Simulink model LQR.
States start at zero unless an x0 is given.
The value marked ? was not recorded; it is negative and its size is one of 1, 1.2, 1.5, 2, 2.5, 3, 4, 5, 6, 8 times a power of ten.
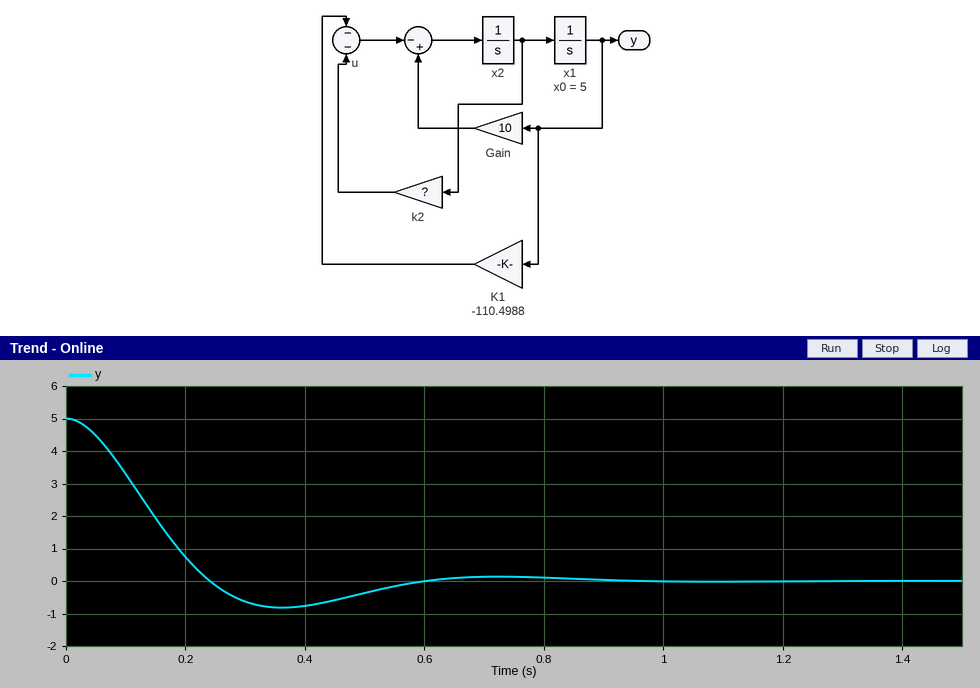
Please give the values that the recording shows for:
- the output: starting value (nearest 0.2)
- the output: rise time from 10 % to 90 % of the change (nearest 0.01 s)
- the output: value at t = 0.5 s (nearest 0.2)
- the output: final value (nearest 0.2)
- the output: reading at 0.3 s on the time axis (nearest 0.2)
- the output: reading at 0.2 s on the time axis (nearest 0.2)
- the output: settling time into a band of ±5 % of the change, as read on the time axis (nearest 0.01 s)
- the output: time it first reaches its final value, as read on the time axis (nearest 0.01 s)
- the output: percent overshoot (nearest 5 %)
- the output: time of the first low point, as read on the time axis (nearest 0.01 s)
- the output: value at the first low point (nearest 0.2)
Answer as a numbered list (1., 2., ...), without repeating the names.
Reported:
1. 5.0
2. 0.16 s
3. -0.4
4. 0.0
5. -0.6
6. 0.8
7. 0.53 s
8. 0.24 s
9. 15 %
10. 0.36 s
11. -0.8
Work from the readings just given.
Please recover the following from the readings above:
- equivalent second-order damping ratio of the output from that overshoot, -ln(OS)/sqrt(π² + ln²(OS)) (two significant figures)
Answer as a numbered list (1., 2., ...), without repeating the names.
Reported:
1. 0.52
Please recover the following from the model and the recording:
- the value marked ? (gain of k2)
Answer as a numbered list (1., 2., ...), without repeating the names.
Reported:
1. -10
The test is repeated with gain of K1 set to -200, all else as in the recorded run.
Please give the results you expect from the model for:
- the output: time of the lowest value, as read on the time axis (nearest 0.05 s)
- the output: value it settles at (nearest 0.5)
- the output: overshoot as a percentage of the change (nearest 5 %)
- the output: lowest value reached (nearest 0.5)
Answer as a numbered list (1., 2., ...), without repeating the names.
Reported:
1. 0.25 s
2. 0.0
3. 30 %
4. -1.5
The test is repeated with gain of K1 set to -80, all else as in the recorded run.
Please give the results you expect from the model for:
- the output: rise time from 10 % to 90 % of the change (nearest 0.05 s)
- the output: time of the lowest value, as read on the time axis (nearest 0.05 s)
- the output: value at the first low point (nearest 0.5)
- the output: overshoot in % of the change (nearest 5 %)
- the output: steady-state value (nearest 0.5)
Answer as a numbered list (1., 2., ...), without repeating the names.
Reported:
1. 0.20 s
2. 0.45 s
3. -0.5
4. 10 %
5. 0.0
